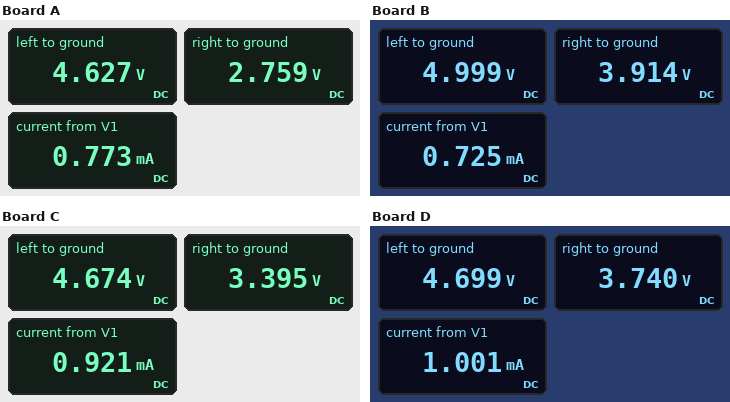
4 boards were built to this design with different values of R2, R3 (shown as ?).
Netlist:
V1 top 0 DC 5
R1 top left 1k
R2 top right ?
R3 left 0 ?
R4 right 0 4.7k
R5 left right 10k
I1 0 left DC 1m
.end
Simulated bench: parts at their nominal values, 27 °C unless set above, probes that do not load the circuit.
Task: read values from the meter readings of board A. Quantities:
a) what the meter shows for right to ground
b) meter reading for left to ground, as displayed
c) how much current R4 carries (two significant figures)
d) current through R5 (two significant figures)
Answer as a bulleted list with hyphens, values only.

- 2.759 V
- 4.627 V
- 590 µA
- 190 µA
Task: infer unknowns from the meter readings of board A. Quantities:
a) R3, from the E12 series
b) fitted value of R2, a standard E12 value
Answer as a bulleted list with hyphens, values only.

- 3.9 kΩ
- 5.6 kΩ
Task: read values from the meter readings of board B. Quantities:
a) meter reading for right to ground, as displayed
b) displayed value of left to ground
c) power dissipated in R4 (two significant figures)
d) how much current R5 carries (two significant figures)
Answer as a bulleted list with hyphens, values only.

- 3.914 V
- 4.999 V
- 3.3 mW
- 110 µA
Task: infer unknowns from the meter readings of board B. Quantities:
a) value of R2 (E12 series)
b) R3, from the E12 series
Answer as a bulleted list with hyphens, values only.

- 1.5 kΩ
- 5.6 kΩ
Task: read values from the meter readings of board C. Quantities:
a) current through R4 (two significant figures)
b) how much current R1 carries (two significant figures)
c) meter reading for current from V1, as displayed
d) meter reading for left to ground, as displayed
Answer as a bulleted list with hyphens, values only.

- 720 µA
- 330 µA
- 0.921 mA
- 4.674 V
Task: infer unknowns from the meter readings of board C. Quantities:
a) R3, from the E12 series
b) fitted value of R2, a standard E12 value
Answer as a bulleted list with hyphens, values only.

- 3.9 kΩ
- 2.7 kΩ
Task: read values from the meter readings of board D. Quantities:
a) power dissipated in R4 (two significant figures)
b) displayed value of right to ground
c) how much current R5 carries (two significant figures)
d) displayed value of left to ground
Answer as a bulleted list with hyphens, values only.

- 3.0 mW
- 3.740 V
- 96 µA
- 4.699 V
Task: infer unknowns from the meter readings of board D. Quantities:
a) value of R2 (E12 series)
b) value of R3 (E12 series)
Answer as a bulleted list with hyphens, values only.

- 1.8 kΩ
- 3.9 kΩ
